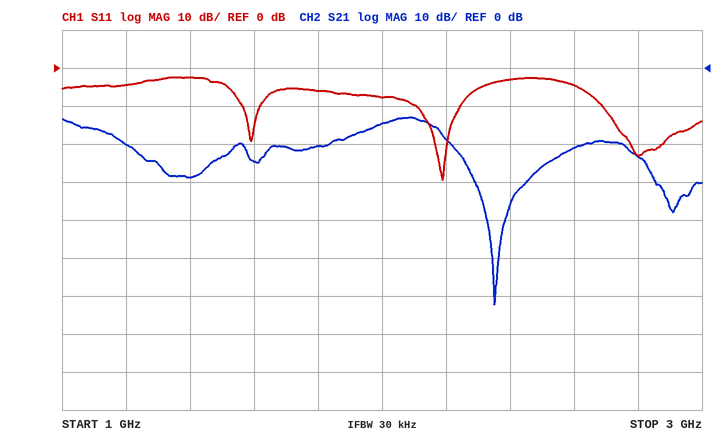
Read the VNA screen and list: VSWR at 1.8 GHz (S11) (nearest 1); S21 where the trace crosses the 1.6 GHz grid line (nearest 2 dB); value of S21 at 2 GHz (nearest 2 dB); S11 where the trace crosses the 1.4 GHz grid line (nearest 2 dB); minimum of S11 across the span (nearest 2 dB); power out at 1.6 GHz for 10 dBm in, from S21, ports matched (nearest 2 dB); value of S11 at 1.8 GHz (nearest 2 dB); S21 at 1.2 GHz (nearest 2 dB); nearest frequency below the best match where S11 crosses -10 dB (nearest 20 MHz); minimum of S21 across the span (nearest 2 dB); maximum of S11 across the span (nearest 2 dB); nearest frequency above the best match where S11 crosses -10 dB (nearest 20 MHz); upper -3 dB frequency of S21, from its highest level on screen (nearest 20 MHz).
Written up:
3
-24 dB
-14 dB
-2 dB
-30 dB
-14 dBm
-6 dB
-20 dB
2.10 GHz
-62 dB
-2 dB
2.24 GHz
2.18 GHz
